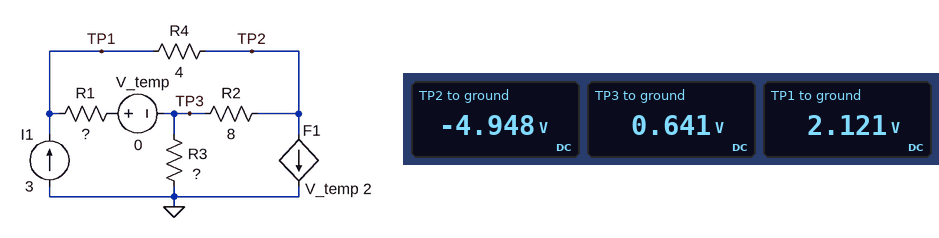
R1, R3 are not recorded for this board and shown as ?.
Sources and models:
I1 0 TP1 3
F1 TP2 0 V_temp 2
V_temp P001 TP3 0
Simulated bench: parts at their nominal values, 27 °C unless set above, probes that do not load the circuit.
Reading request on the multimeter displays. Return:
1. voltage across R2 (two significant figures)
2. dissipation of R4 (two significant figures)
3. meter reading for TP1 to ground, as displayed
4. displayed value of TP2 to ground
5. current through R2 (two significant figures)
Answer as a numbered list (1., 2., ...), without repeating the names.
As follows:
1. 5.6 V
2. 12 W
3. 2.121 V
4. -4.948 V
5. 700 mA
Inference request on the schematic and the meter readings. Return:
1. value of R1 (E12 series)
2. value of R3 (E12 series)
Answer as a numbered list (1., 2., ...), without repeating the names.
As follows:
1. 1.2 Ω
2. 1.2 Ω
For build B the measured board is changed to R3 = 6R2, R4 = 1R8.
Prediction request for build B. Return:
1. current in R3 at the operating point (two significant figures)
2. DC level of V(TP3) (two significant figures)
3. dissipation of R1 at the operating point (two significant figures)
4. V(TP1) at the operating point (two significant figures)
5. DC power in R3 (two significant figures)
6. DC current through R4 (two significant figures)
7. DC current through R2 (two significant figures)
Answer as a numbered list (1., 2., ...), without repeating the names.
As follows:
1. 820 mA
2. 5.1 V
3. 1.4 W
4. 6.4 V
5. 4.2 W
6. 1.9 A
7. 270 mA
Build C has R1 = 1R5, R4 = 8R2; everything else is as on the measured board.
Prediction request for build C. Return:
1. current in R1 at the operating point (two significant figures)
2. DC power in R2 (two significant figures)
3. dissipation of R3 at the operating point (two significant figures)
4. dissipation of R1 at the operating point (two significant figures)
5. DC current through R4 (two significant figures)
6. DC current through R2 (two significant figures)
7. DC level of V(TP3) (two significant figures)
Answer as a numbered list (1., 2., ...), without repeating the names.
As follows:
1. 1.4 A
2. 14 W
3. 16 mW
4. 3.1 W
5. 1.6 A
6. 1.3 A
7. 140 mV
